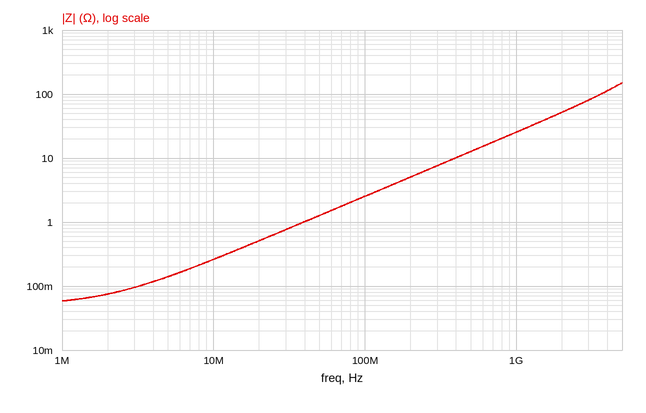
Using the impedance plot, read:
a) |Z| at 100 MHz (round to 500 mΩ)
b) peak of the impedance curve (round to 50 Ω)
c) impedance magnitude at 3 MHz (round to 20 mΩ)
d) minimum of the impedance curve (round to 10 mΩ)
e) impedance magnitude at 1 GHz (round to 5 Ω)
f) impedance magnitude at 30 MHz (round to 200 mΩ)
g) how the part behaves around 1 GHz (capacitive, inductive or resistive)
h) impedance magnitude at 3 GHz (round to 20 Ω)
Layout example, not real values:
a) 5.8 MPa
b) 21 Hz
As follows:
a) 2.5 Ω
b) 150 Ω
c) 100 mΩ
d) 60 mΩ
e) 25 Ω
f) 800 mΩ
g) inductive
h) 80 Ω
